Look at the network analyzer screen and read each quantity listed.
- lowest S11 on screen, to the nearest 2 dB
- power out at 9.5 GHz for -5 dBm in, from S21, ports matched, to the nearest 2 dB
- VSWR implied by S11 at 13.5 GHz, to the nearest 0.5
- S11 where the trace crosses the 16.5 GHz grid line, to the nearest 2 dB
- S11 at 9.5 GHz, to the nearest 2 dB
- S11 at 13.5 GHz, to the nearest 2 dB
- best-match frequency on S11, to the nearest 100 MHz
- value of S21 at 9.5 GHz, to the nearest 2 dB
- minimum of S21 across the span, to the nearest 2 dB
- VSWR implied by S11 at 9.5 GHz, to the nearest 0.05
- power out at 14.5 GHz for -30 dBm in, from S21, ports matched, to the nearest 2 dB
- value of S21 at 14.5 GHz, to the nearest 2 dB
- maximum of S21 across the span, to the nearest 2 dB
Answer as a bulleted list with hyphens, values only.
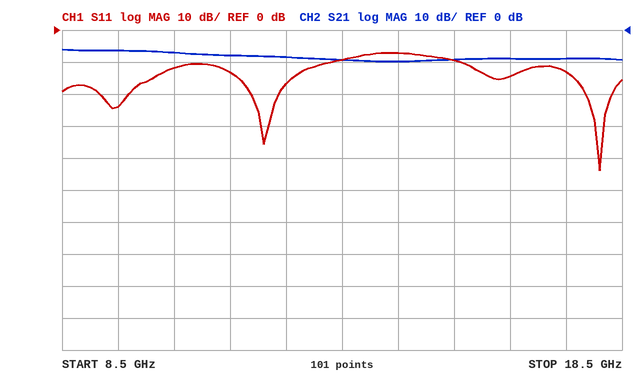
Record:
- -44 dB
- -12 dBm
- 2.0
- -14 dB
- -24 dB
- -10 dB
- 18.1 GHz
- -6 dB
- -10 dB
- 1.15
- -40 dBm
- -10 dB
- -6 dB
